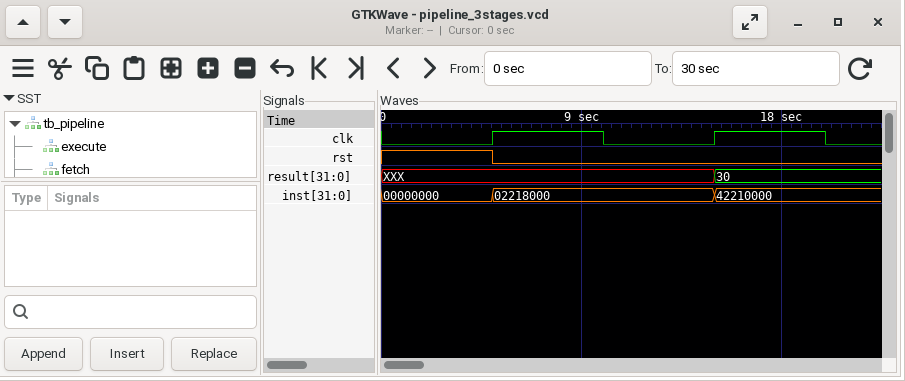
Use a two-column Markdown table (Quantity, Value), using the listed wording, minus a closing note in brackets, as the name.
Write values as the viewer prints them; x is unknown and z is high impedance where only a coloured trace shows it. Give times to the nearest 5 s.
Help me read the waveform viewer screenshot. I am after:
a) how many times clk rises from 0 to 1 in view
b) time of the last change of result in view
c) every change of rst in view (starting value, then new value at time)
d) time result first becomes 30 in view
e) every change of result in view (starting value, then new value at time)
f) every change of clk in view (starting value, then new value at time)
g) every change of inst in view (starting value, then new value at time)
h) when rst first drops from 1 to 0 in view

| Quantity | Value |
|---|---|
| how many times clk rises from 0 to 1 in view | 2 |
| time of the last change of result in view | 15 s |
| every change of rst in view | 1, 0 at 5 s |
| time result first becomes 30 in view | 15 s |
| every change of result in view | XXX, 30 at 15 s |
| every change of clk in view | 0, 1 at 5 s, 0 at 10 s, 1 at 15 s, 0 at 20 s |
| every change of inst in view | 00000000, 02218000 at 5 s, 42210000 at 15 s |
| when rst first drops from 1 to 0 in view | 5 s |
